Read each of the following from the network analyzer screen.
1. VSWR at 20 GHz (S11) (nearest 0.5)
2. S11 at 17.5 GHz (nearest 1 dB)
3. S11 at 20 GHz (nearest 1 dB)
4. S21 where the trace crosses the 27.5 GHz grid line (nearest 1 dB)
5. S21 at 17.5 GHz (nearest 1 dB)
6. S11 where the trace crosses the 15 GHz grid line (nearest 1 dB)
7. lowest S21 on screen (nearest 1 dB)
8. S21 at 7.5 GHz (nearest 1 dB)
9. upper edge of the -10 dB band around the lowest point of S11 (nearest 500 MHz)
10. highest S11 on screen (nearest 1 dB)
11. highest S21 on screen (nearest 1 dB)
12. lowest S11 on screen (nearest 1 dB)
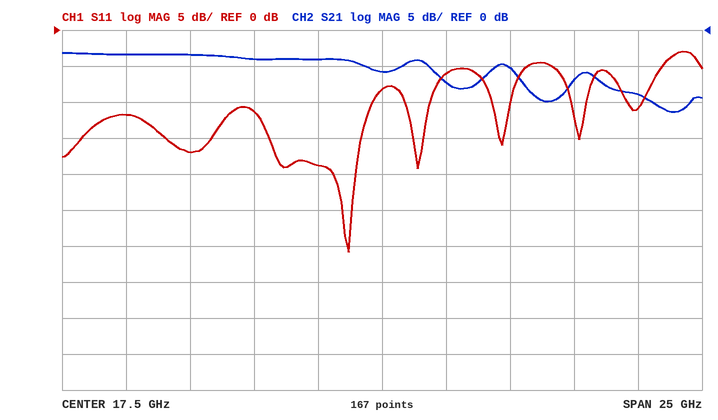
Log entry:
3.0
-8 dB
-6 dB
-9 dB
-6 dB
-19 dB
-11 dB
-3 dB
17.0 GHz
-3 dB
-3 dB
-31 dB
